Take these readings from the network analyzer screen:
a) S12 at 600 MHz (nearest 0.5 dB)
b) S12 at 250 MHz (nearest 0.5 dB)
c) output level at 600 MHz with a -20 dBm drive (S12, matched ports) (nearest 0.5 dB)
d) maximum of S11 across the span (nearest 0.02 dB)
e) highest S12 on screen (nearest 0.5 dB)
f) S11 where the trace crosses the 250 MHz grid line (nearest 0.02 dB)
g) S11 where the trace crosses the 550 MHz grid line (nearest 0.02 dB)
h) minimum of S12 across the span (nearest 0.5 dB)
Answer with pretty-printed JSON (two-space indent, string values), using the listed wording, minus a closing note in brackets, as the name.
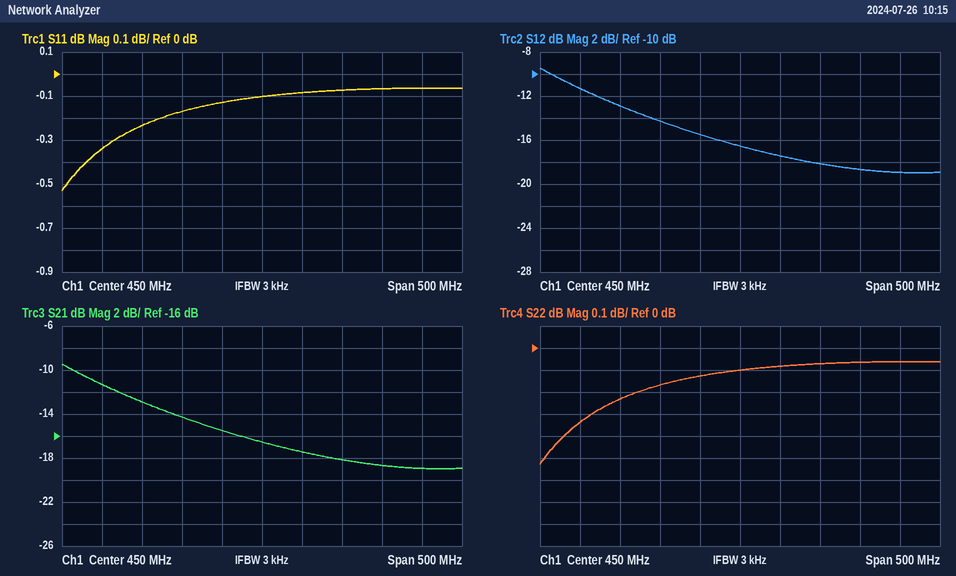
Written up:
{
  "S12 at 600 MHz": "-18.5 dB",
  "S12 at 250 MHz": "-11.5 dB",
  "output level at 600 MHz with a -20 dBm drive (S12, matched ports)": "-38.5 dBm",
  "maximum of S11 across the span": "-0.06 dB",
  "highest S12 on screen": "-9.5 dB",
  "S11 where the trace crosses the 250 MHz grid line": "-0.34 dB",
  "S11 where the trace crosses the 550 MHz grid line": "-0.08 dB",
  "minimum of S12 across the span": "-19.0 dB"
}
